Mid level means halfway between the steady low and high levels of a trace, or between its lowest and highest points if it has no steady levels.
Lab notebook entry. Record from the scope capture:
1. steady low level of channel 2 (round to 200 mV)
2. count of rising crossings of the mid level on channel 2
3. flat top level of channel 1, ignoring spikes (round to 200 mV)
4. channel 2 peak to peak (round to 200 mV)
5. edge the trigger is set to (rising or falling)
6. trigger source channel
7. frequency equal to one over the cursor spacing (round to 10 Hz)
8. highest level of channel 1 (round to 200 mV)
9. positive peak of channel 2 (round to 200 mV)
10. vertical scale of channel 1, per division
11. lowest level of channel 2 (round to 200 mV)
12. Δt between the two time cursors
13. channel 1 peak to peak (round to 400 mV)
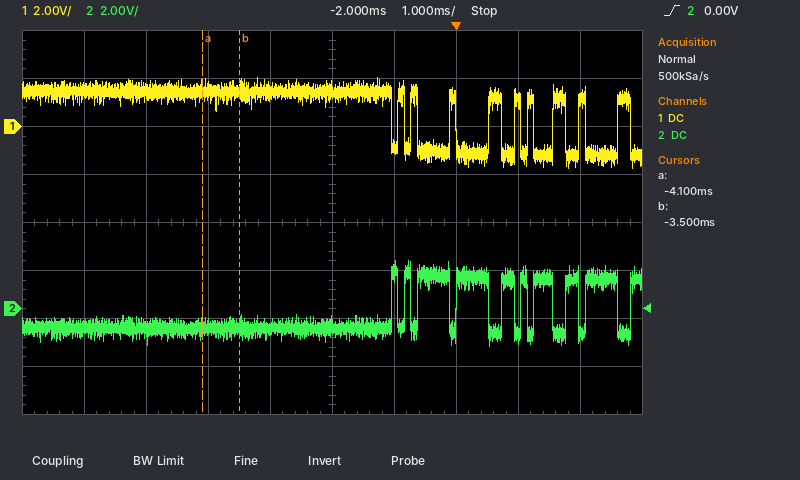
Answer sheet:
-800 mV
10
1.4 V
3.6 V
rising
channel 2
1.67 kHz
2.0 V
2.0 V
2 V
-1.6 V
600 µs
3.6 V
